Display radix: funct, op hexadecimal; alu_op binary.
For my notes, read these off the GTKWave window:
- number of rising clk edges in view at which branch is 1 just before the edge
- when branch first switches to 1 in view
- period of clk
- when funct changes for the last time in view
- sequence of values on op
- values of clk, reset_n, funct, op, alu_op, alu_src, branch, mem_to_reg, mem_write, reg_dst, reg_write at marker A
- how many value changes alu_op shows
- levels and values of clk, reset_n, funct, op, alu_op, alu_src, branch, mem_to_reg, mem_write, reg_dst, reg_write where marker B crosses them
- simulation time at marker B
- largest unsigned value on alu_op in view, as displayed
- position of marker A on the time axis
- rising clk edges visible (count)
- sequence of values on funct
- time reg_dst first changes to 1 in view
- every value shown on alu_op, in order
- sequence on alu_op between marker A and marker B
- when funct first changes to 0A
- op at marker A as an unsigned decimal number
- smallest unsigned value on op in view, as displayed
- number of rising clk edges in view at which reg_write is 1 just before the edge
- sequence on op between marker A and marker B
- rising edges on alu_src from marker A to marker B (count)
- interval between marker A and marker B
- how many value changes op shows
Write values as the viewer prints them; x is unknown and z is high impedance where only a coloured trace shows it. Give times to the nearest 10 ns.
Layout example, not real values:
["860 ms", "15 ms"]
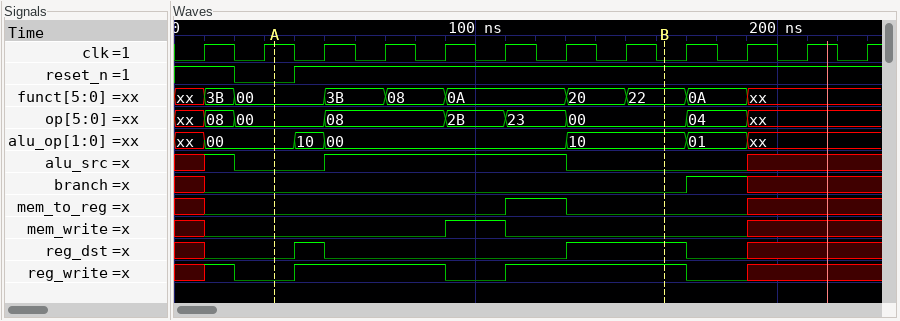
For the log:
["1", "170 ns", "20 ns", "190 ns", "xx, 08, 00, 08, 2B, 23, 00, 04, xx", "clk=1, reset_n=0, funct=00, op=00, alu_op=00, alu_src=0, branch=0, mem_to_reg=0, mem_write=0, reg_dst=0, reg_write=0", "6", "clk=0, reset_n=1, funct=22, op=00, alu_op=10, alu_src=0, branch=0, mem_to_reg=0, mem_write=0, reg_dst=1, reg_write=1", "160 ns", "10", "30 ns", "12", "xx, 3B, 00, 3B, 08, 0A, 20, 22, 0A, xx", "40 ns", "xx, 00, 10, 00, 10, 01, xx", "00, 10, 00, 10", "90 ns", "0", "00", "6", "00, 08, 2B, 23, 00", "1", "130 ns", "8"]
